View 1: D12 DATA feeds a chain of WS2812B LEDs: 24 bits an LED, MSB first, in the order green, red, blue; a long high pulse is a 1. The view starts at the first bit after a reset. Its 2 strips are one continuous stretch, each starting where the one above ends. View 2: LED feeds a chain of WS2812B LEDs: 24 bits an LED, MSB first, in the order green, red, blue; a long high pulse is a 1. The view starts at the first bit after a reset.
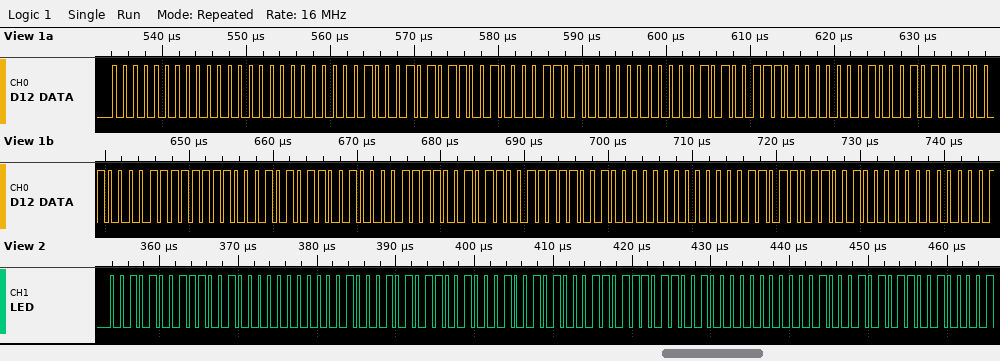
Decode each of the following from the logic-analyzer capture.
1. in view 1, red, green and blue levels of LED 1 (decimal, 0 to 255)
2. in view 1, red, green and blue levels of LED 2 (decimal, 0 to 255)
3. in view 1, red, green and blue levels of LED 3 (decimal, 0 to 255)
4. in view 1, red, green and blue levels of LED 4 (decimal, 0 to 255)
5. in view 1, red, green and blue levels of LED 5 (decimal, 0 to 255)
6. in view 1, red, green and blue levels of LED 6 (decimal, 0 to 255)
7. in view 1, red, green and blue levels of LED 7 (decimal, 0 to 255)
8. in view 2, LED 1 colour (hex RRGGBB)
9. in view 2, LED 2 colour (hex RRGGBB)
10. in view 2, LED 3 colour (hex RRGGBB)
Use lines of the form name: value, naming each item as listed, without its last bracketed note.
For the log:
in view 1, red, green and blue levels of LED 1: 0, 0, 0
in view 1, red, green and blue levels of LED 2: 200, 138, 104
in view 1, red, green and blue levels of LED 3: 167, 0, 0
in view 1, red, green and blue levels of LED 4: 200, 138, 127
in view 1, red, green and blue levels of LED 5: 200, 138, 121
in view 1, red, green and blue levels of LED 6: 200, 103, 0
in view 1, red, green and blue levels of LED 7: 200, 54, 0
in view 2, LED 1 colour: #C82900
in view 2, LED 2 colour: #C88A94
in view 2, LED 3 colour: #C86E00
